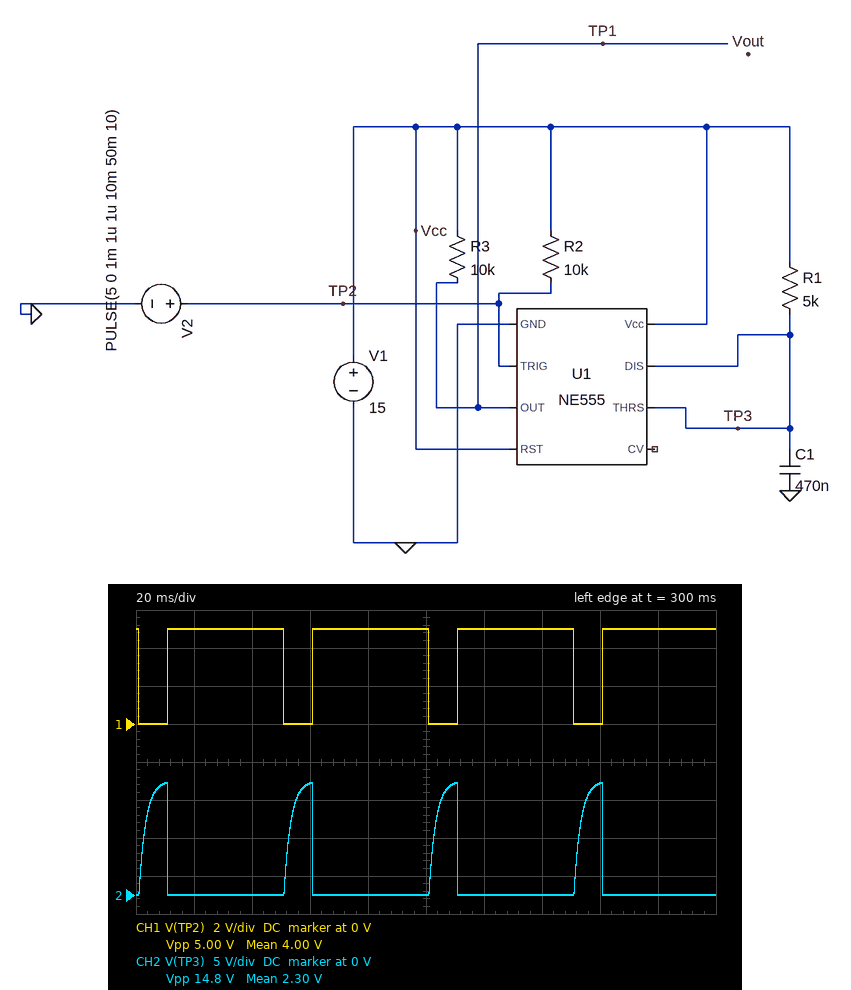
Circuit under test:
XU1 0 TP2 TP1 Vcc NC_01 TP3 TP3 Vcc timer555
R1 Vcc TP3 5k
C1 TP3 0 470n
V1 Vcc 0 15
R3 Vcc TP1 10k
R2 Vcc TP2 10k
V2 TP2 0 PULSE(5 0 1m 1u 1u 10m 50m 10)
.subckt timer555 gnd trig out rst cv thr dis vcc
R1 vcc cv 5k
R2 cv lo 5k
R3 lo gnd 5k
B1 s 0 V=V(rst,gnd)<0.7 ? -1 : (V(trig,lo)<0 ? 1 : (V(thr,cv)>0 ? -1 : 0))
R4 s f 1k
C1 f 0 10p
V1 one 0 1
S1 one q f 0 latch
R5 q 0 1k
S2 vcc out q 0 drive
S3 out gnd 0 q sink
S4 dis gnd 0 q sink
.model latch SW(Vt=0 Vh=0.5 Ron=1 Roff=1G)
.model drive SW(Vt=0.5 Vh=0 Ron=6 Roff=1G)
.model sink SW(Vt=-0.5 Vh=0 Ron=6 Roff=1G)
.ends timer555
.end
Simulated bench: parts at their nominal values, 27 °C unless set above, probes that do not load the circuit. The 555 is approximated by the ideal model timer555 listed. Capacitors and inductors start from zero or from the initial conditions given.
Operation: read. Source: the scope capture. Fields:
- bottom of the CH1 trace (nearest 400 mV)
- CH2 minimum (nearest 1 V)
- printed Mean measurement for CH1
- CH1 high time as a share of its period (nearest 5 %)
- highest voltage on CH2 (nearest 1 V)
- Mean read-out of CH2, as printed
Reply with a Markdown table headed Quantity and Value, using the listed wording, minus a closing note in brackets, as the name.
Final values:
| Quantity | Value |
|---|---|
| bottom of the CH1 trace | 0 V |
| CH2 minimum | 0 V |
| printed Mean measurement for CH1 | 4.00 V |
| CH1 high time as a share of its period | 80 % |
| highest voltage on CH2 | 15 V |
| Mean read-out of CH2, as printed | 2.30 V |
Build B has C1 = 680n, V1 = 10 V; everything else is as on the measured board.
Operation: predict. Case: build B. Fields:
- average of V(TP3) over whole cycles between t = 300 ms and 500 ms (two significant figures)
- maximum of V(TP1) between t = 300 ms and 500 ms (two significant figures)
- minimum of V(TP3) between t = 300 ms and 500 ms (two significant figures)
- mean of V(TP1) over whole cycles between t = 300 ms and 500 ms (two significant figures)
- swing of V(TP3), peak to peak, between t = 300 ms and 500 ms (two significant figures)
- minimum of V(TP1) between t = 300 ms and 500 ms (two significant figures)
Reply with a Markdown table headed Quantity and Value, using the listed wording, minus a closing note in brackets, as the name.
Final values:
| Quantity | Value |
|---|---|
| average of V(TP3) over whole cycles between t = 300 ms and 500 ms | 1.4 V |
| maximum of V(TP1) between t = 300 ms and 500 ms | 10 V |
| minimum of V(TP3) between t = 300 ms and 500 ms | 12 mV |
| mean of V(TP1) over whole cycles between t = 300 ms and 500 ms | 2.0 V |
| swing of V(TP3), peak to peak, between t = 300 ms and 500 ms | 9.5 V |
| minimum of V(TP1) between t = 300 ms and 500 ms | 6.0 mV |
